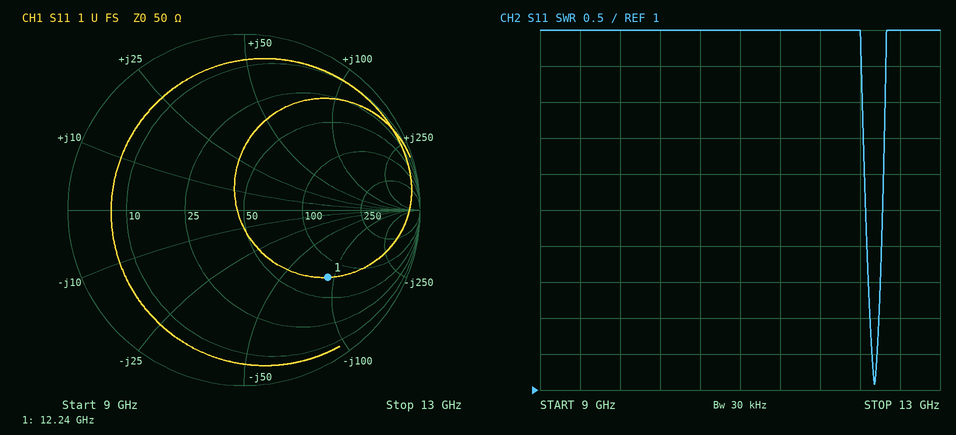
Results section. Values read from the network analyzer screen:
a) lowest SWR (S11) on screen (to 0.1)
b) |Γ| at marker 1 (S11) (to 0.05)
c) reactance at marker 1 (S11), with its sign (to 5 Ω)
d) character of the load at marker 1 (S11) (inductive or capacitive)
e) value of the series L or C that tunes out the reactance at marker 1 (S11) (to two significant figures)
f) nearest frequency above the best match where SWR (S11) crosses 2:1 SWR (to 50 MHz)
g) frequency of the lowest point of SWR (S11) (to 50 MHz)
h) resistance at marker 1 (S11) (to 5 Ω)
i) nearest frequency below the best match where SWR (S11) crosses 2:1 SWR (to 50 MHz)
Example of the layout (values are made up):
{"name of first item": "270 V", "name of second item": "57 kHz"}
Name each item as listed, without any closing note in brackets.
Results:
{"lowest SWR (S11) on screen": "1.1", "|Γ| at marker 1 (S11)": "0.60", "reactance at marker 1 (S11), with its sign": "-90 Ω", "character of the load at marker 1 (S11)": "capacitive", "value of the series L or C that tunes out the reactance at marker 1 (S11)": "1.2 nH", "nearest frequency above the best match where SWR (S11) crosses 2:1 SWR": "12.40 GHz", "frequency of the lowest point of SWR (S11)": "12.35 GHz", "resistance at marker 1 (S11)": "75 Ω", "nearest frequency below the best match where SWR (S11) crosses 2:1 SWR": "12.30 GHz"}
